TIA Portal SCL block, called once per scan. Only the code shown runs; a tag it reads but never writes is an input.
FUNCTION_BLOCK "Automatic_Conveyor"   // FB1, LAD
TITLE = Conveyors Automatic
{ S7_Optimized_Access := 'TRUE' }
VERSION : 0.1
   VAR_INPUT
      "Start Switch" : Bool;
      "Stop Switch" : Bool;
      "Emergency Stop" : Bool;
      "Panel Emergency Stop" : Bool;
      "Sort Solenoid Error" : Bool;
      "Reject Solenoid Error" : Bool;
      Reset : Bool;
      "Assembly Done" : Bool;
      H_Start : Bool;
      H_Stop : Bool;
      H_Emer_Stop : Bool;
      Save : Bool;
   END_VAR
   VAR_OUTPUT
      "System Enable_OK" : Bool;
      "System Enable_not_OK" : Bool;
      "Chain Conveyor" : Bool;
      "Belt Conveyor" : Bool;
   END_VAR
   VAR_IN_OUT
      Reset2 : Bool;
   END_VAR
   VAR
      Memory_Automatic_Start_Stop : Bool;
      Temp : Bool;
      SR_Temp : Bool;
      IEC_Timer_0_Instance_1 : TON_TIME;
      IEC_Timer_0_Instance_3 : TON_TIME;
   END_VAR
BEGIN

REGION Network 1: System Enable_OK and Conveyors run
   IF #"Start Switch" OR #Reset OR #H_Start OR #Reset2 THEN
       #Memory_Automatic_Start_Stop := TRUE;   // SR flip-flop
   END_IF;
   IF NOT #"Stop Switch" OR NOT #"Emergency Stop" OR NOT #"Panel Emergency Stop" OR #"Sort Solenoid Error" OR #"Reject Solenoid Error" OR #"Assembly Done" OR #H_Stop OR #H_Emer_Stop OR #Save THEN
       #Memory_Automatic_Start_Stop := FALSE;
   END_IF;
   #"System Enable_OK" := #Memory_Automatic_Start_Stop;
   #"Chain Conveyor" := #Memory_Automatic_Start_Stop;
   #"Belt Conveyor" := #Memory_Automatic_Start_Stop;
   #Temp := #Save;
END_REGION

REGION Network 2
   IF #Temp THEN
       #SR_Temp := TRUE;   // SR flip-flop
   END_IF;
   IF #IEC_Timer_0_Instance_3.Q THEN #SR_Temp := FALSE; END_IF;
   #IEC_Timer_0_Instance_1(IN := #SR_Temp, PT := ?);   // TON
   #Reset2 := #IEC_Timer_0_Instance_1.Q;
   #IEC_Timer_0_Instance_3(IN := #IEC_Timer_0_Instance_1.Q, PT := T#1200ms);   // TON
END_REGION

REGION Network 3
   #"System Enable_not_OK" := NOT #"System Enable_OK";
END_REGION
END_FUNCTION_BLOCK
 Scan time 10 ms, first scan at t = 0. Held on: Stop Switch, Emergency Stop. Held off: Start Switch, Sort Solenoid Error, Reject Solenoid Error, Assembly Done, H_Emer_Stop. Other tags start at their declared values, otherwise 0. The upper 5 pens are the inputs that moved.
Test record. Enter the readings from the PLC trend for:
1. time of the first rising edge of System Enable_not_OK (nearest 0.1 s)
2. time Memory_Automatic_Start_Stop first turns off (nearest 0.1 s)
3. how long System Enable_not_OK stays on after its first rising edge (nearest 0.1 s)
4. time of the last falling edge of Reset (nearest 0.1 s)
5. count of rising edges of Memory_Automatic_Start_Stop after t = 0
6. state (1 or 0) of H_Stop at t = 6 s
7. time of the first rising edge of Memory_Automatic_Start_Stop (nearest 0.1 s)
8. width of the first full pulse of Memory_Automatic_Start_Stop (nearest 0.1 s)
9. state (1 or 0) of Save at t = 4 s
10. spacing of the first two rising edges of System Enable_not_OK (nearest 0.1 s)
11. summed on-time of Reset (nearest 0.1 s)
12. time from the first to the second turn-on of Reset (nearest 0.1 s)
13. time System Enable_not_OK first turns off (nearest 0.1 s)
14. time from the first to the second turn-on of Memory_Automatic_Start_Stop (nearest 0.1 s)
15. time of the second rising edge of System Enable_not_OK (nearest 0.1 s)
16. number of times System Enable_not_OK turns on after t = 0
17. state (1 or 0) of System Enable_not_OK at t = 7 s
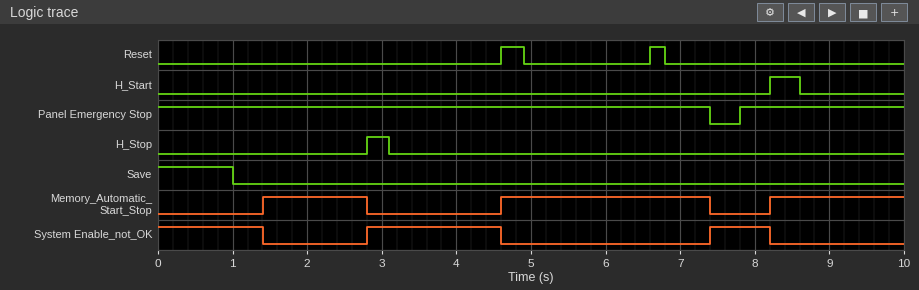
2.8 s
2.8 s
1.8 s
6.8 s
3
0
1.4 s
1.4 s
0
4.6 s
0.5 s
2.0 s
1.4 s
3.2 s
7.4 s
2
0
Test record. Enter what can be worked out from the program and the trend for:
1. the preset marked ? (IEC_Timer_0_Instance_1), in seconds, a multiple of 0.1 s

1.4 s
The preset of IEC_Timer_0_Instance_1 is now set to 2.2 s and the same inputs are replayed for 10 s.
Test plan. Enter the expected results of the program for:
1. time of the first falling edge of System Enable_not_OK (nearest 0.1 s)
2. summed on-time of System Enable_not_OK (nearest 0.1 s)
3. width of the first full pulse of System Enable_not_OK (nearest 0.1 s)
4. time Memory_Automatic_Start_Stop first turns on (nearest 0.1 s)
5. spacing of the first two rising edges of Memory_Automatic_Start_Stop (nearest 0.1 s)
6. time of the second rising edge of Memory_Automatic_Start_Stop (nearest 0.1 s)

2.2 s
3.3 s
0.3 s
2.2 s
0.9 s
3.1 s
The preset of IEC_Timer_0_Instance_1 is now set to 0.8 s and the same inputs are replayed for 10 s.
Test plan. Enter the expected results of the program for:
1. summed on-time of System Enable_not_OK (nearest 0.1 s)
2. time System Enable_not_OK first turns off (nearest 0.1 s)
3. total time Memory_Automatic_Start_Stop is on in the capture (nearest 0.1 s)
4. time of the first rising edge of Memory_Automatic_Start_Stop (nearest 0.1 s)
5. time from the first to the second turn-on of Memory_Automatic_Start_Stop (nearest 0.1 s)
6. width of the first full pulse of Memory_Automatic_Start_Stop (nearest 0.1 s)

3.6 s
1.0 s
6.4 s
1.0 s
3.6 s
1.8 s
